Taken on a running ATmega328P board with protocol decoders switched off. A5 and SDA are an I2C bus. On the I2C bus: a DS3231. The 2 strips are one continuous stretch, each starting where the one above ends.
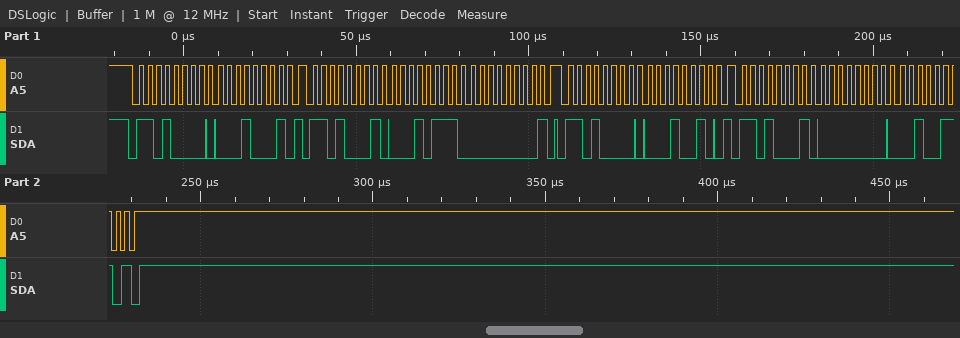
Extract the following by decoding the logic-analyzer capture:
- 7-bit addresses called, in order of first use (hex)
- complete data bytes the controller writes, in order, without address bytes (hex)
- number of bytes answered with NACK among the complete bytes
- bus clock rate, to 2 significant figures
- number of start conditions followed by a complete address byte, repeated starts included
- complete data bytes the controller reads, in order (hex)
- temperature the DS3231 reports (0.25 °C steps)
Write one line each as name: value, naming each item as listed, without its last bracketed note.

7-bit addresses called, in order of first use: 0x68
complete data bytes the controller writes, in order, without address bytes: 11 12
number of bytes answered with NACK among the complete bytes: 2
bus clock rate, to 2 significant figures: 400 kHz
number of start conditions followed by a complete address byte, repeated starts included: 4
complete data bytes the controller reads, in order: 17 00 00 26
temperature the DS3231 reports: 23.00 °C
